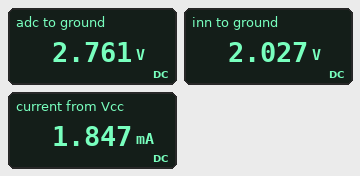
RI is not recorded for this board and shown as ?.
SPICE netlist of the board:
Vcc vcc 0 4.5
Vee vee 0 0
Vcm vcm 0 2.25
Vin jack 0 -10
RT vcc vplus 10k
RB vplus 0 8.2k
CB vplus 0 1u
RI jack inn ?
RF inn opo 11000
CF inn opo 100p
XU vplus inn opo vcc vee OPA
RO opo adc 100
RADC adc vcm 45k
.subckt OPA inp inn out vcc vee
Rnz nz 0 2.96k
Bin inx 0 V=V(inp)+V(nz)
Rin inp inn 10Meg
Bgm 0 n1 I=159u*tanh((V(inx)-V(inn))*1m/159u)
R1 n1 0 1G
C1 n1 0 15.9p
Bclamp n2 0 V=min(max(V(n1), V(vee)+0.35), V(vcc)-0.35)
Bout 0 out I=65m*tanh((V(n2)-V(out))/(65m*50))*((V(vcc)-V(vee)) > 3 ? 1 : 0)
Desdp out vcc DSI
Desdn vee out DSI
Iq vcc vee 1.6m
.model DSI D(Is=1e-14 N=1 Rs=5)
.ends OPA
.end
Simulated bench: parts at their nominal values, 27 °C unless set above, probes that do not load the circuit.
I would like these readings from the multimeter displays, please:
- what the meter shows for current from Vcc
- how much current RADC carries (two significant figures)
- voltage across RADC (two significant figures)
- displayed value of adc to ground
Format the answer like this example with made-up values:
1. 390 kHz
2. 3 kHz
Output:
1. 1.847 mA
2. 11 µA
3. 510 mV
4. 2.761 V
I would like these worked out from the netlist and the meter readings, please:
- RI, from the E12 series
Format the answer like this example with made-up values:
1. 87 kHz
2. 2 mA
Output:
1. 180 kΩ
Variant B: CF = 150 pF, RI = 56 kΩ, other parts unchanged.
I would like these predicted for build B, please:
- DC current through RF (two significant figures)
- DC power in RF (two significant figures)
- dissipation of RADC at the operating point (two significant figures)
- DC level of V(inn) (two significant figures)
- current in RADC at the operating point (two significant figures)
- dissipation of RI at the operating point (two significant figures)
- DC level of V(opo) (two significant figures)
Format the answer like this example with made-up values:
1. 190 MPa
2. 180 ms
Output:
1. 210 µA
2. 490 µW
3. 79 µW
4. 1.8 V
5. 42 µA
6. 2.5 mW
7. 4.1 V
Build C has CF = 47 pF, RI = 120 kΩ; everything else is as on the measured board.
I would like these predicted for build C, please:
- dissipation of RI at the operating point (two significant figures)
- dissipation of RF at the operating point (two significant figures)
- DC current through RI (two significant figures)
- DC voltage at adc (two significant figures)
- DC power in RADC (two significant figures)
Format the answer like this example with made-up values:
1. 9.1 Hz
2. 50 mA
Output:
1. 1.2 mW
2. 110 µW
3. 100 µA
4. 3.1 V
5. 17 µW
